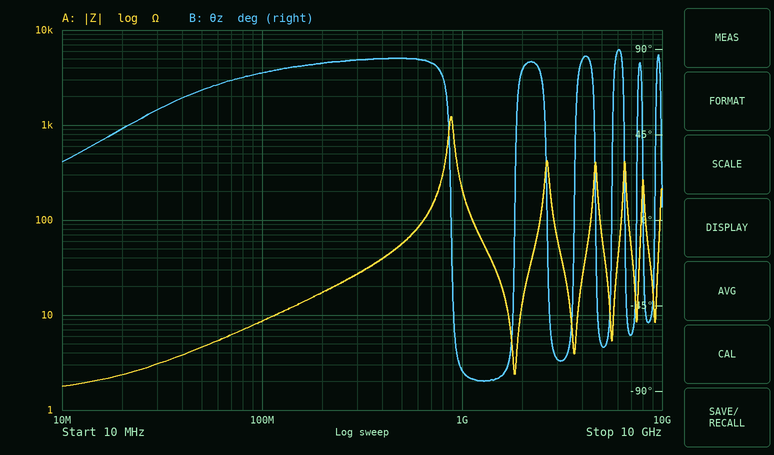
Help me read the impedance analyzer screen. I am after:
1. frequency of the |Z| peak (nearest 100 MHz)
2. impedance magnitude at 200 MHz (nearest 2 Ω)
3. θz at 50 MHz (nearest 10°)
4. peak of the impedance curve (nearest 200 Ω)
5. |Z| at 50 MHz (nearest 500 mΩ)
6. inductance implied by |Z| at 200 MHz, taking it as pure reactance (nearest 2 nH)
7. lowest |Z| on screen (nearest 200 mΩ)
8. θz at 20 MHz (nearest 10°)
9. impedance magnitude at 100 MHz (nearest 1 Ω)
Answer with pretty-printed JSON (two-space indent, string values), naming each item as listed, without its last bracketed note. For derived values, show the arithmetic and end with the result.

{
  "frequency of the |Z| peak": "900 MHz",
  "impedance magnitude at 200 MHz": "18 Ω",
  "θz at 50 MHz": "70°",
  "peak of the impedance curve": "1.2 kΩ",
  "|Z| at 50 MHz": "4.5 Ω",
  "inductance implied by |Z| at 200 MHz, taking it as pure reactance": "L = 18 Ω/(2π × 200 MHz) ≈ 14 nH",
  "lowest |Z| on screen": "1.8 Ω",
  "θz at 20 MHz": "50°",
  "impedance magnitude at 100 MHz": "9 Ω"
}
